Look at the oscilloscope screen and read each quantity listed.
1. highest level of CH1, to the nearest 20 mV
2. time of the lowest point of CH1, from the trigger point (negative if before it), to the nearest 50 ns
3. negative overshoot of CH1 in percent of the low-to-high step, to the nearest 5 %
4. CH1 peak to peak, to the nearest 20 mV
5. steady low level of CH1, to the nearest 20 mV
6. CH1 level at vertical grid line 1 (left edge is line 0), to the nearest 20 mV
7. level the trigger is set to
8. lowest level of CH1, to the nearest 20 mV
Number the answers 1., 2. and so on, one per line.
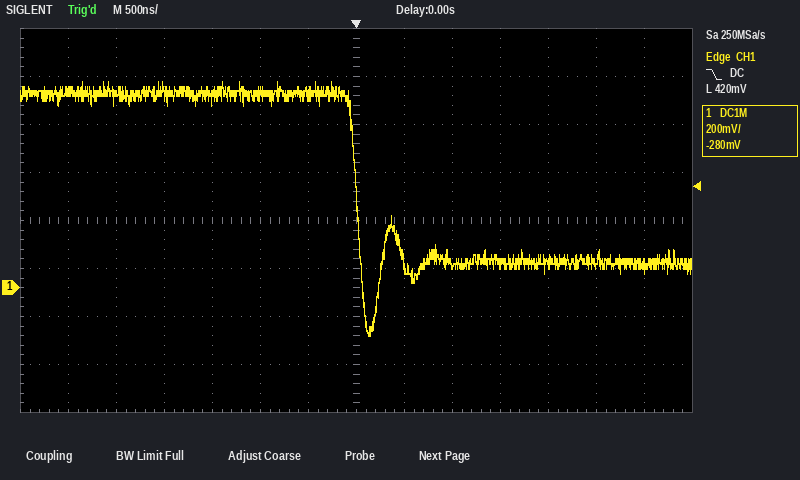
1. 860 mV
2. +150 ns
3. 45 %
4. 1.06 V
5. 100 mV
6. 820 mV
7. 420 mV
8. -200 mV
